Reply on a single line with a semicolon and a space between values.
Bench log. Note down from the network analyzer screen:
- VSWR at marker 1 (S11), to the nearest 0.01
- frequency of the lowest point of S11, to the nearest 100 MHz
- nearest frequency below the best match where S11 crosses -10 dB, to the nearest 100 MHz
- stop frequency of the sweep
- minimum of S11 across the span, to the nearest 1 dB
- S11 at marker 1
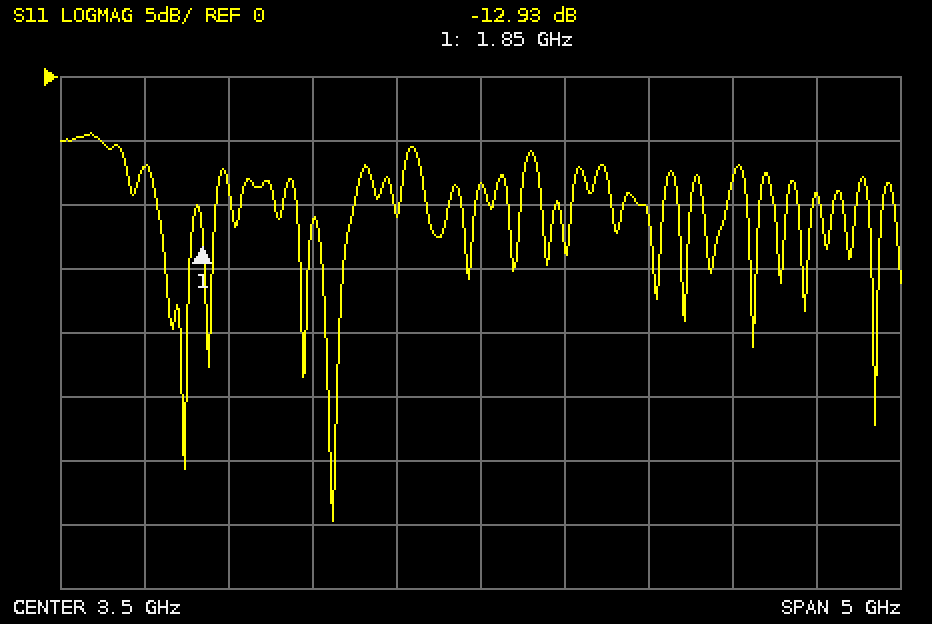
1.58; 2.6 GHz; 2.4 GHz; 6 GHz; -35 dB; -12.93 dB
